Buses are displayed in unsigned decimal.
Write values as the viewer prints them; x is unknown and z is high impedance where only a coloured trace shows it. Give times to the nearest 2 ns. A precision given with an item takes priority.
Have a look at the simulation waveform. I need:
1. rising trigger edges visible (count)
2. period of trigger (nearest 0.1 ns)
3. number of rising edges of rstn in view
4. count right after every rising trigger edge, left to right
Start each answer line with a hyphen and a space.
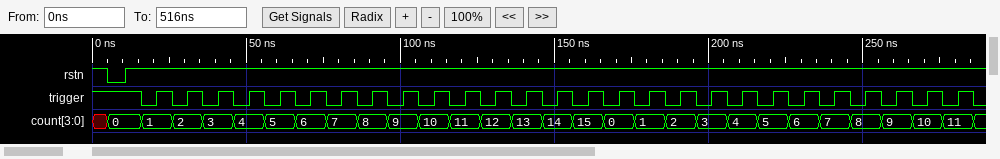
- 27
- 10 ns
- 1
- 1, 2, 3, 4, 5, 6, 7, 8, 9, 10, 11, 12, 13, 14, 15, 0, 1, 2, 3, 4, 5, 6, 7, 8, 9, 10, 11
